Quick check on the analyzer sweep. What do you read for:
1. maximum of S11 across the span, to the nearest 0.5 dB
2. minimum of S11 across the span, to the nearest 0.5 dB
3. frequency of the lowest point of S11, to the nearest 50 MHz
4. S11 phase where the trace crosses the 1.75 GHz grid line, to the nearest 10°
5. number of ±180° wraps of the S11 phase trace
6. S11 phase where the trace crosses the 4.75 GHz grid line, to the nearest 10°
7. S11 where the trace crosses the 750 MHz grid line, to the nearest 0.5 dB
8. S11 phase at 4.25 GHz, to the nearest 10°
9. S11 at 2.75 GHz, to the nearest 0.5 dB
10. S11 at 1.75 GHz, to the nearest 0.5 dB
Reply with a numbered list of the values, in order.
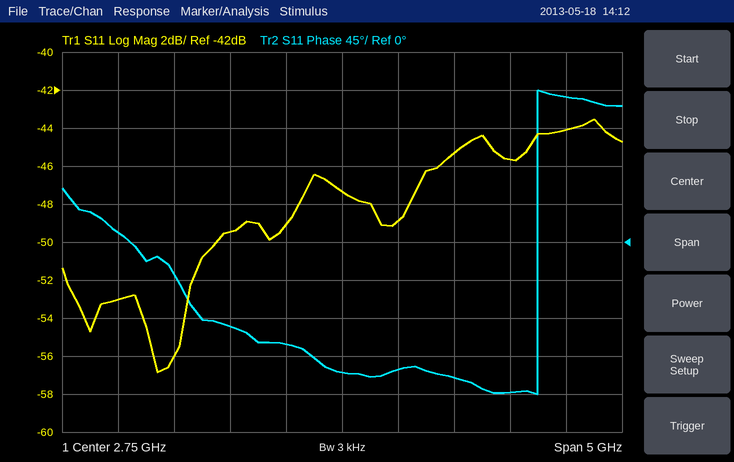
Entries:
1. -43.5 dB
2. -57.0 dB
3. 1.10 GHz
4. -100°
5. 1
6. 170°
7. -53.0 dB
8. -180°
9. -47.5 dB
10. -49.5 dB
